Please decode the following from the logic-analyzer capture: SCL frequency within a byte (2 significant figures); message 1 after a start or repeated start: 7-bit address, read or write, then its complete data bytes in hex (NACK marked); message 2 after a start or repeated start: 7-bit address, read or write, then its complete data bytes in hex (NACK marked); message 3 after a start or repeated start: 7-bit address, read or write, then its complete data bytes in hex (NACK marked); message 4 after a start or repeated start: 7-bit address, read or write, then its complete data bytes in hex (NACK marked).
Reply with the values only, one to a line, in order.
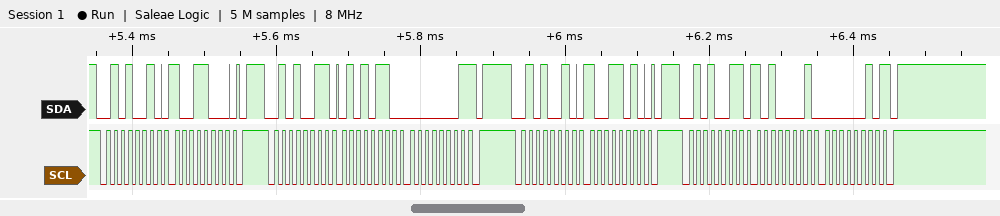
100 kHz
0x29 write: 98
0x29 read: 56 01 NACK
0x29 write: 9A
0x29 read: A1 02 NACK
